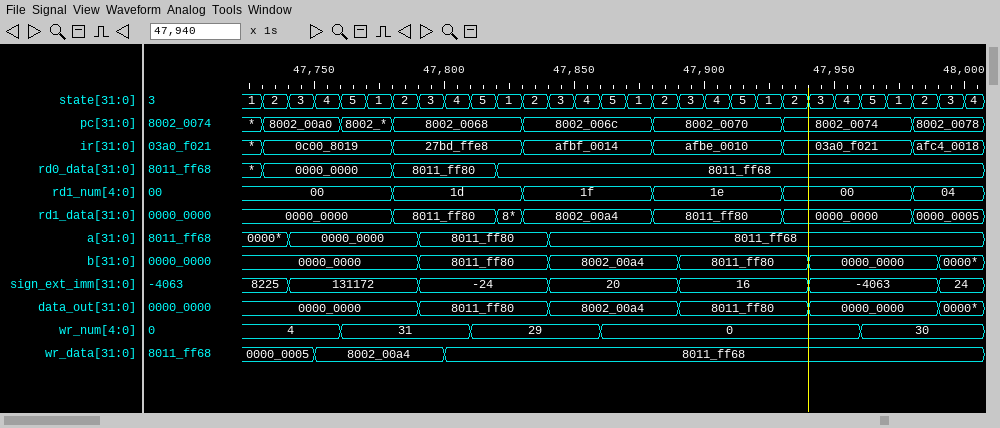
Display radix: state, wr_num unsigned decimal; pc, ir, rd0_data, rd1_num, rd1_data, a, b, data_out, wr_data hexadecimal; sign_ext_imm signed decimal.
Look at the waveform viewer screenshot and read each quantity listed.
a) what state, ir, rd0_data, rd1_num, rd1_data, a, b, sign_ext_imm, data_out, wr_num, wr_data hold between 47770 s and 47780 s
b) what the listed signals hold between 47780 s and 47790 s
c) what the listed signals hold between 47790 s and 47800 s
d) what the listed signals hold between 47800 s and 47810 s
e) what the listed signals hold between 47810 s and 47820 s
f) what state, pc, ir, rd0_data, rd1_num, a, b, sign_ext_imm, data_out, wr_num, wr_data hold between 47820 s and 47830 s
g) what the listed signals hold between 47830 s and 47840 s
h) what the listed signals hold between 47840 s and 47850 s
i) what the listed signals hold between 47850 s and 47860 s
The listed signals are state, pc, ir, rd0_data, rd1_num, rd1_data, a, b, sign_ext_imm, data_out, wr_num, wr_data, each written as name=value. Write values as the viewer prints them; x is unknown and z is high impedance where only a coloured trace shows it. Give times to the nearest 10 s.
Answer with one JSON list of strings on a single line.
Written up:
["state=1, ir=0c00_8019, rd0_data=0000_0000, rd1_num=00, rd1_data=0000_0000, a=0000_0000, b=0000_0000, sign_ext_imm=131172, data_out=0000_0000, wr_num=31, wr_data=8002_00a4", "state=2, pc=8002_0068, ir=27bd_ffe8, rd0_data=8011_ff80, rd1_num=1d, rd1_data=8011_ff80, a=0000_0000, b=0000_0000, sign_ext_imm=131172, data_out=0000_0000, wr_num=31, wr_data=8002_00a4", "state=3, pc=8002_0068, ir=27bd_ffe8, rd0_data=8011_ff80, rd1_num=1d, rd1_data=8011_ff80, a=8011_ff80, b=8011_ff80, sign_ext_imm=-24, data_out=8011_ff80, wr_num=31, wr_data=8002_00a4", "state=4, pc=8002_0068, ir=27bd_ffe8, rd0_data=8011_ff80, rd1_num=1d, rd1_data=8011_ff80, a=8011_ff80, b=8011_ff80, sign_ext_imm=-24, data_out=8011_ff80, wr_num=31, wr_data=8011_ff68", "state=5, pc=8002_0068, ir=27bd_ffe8, rd0_data=8011_ff80, rd1_num=1d, rd1_data=8011_ff80, a=8011_ff80, b=8011_ff80, sign_ext_imm=-24, data_out=8011_ff80, wr_num=29, wr_data=8011_ff68", "state=1, pc=8002_0068, ir=27bd_ffe8, rd0_data=8011_ff68, rd1_num=1d, a=8011_ff80, b=8011_ff80, sign_ext_imm=-24, data_out=8011_ff80, wr_num=29, wr_data=8011_ff68", "state=2, pc=8002_006c, ir=afbf_0014, rd0_data=8011_ff68, rd1_num=1f, rd1_data=8002_00a4, a=8011_ff80, b=8011_ff80, sign_ext_imm=-24, data_out=8011_ff80, wr_num=29, wr_data=8011_ff68", "state=3, pc=8002_006c, ir=afbf_0014, rd0_data=8011_ff68, rd1_num=1f, rd1_data=8002_00a4, a=8011_ff68, b=8002_00a4, sign_ext_imm=20, data_out=8002_00a4, wr_num=29, wr_data=8011_ff68", "state=4, pc=8002_006c, ir=afbf_0014, rd0_data=8011_ff68, rd1_num=1f, rd1_data=8002_00a4, a=8011_ff68, b=8002_00a4, sign_ext_imm=20, data_out=8002_00a4, wr_num=29, wr_data=8011_ff68"]
